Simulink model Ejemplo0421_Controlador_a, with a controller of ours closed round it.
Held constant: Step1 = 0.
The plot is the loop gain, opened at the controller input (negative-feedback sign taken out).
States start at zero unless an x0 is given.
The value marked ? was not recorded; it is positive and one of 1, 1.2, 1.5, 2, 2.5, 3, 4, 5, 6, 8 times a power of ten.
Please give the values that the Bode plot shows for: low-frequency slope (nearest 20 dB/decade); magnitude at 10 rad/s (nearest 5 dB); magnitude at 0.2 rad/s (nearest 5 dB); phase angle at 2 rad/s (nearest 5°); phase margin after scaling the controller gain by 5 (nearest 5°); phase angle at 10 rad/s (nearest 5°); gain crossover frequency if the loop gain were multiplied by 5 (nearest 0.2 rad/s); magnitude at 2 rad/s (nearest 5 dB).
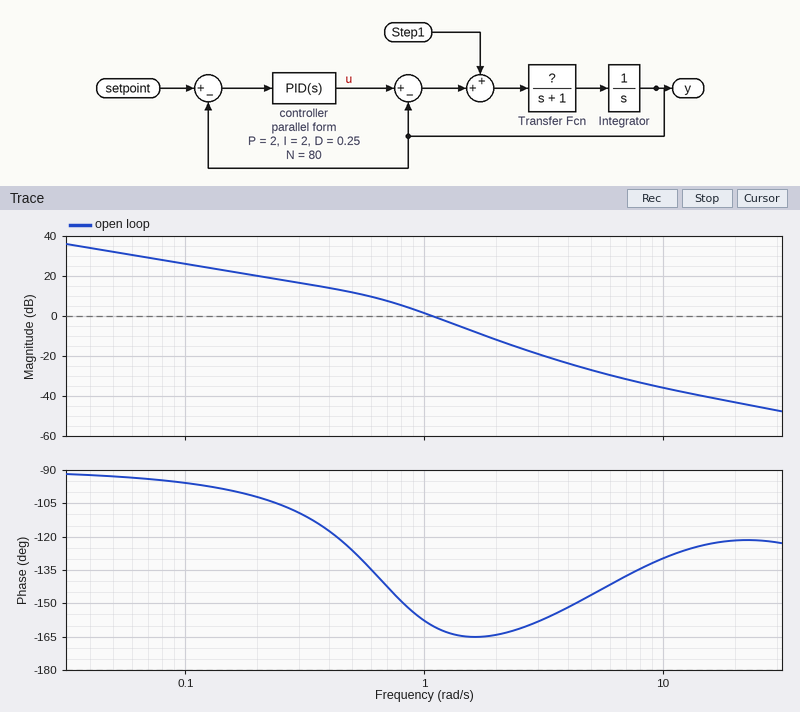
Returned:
-20 dB/decade
-35 dB
20 dB
-165°
15°
-130°
2.2 rad/s
-10 dB
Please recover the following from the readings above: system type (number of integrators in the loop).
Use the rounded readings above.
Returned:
1
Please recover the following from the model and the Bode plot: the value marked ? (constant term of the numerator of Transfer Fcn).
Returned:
0.5
